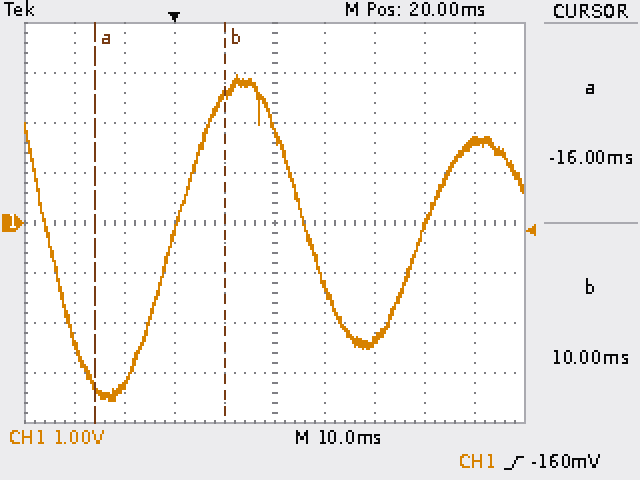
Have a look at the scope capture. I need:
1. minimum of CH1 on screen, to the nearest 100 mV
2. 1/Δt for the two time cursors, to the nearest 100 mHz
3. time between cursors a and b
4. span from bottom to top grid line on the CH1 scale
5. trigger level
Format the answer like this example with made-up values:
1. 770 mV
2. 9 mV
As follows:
1. -3.6 V
2. 38.5 Hz
3. 26 ms
4. 8 V
5. -160 mV
